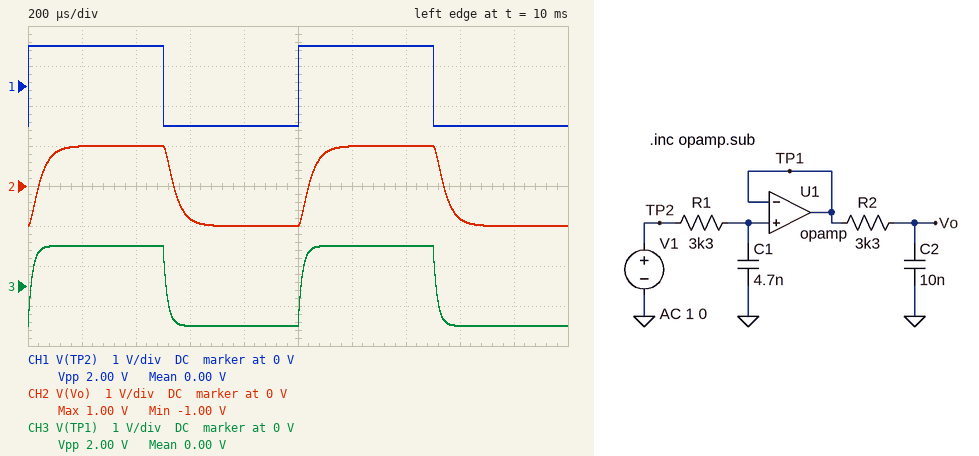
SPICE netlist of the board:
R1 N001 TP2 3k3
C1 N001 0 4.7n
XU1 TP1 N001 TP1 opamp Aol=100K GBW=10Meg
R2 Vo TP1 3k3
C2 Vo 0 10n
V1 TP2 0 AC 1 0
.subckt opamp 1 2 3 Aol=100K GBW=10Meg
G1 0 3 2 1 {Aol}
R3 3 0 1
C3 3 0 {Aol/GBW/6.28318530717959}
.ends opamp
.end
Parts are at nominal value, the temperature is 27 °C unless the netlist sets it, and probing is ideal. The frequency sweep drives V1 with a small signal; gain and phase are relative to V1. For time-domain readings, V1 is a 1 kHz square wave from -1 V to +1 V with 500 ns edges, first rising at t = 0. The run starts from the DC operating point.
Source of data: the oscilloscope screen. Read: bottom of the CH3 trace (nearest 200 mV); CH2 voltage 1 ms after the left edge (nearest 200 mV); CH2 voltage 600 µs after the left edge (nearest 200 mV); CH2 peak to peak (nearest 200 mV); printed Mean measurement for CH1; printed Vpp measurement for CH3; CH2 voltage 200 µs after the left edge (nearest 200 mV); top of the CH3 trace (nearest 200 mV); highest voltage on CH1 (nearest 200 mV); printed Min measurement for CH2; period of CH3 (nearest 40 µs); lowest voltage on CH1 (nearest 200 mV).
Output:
-1.0 V
-1.0 V
-800 mV
2.0 V
0.00 V
2.00 V
1.0 V
1.0 V
1.0 V
-1.00 V
1.00 ms
-1.0 V
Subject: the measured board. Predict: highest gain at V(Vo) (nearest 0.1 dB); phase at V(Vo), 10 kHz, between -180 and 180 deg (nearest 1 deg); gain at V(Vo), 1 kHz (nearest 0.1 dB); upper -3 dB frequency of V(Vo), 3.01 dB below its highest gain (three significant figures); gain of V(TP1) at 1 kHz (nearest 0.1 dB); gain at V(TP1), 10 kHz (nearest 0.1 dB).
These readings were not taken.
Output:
0 dB
-109 deg
-0.2 dB
4.10 kHz
0 dB
-2.9 dB
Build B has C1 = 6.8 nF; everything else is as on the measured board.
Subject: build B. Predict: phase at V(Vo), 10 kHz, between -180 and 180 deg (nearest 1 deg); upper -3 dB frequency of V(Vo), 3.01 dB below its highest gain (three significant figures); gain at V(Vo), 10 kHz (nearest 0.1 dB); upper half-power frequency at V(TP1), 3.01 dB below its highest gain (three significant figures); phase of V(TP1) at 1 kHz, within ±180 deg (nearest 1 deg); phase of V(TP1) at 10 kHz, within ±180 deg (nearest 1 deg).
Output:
-119 deg
3.67 kHz
-12.0 dB
7.09 kHz
-8 deg
-55 deg
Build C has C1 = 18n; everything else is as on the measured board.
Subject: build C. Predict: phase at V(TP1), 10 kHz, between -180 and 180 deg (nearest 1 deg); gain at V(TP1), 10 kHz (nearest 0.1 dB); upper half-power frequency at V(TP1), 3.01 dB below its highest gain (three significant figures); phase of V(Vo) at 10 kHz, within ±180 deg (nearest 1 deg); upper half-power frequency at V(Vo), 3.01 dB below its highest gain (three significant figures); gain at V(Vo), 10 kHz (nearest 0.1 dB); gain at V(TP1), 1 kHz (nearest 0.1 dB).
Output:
-75 deg
-11.7 dB
2.68 kHz
-139 deg
2.18 kHz
-19.0 dB
-0.6 dB
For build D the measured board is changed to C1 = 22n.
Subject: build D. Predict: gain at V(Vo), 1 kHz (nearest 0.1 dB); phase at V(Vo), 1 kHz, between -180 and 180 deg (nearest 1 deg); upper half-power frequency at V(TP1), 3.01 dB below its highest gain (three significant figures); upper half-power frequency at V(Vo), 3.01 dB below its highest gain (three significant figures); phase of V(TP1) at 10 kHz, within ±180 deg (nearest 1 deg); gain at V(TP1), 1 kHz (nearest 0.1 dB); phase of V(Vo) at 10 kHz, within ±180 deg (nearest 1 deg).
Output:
-1.0 dB
-36 deg
2.19 kHz
1.88 kHz
-78 deg
-0.8 dB
-142 deg
